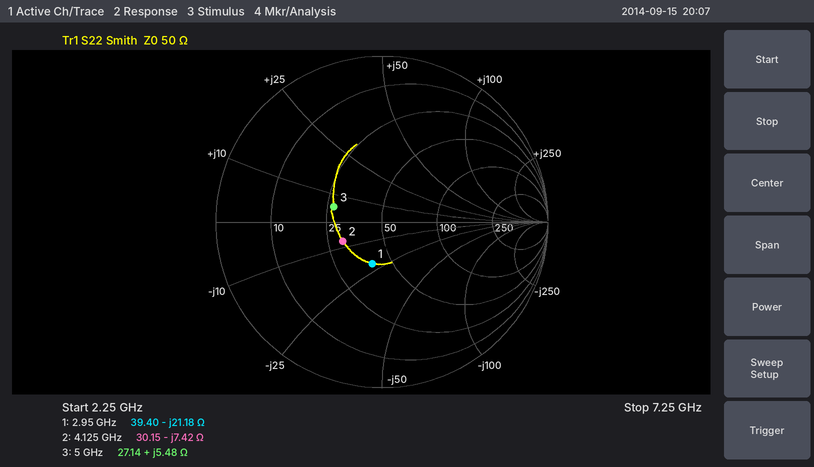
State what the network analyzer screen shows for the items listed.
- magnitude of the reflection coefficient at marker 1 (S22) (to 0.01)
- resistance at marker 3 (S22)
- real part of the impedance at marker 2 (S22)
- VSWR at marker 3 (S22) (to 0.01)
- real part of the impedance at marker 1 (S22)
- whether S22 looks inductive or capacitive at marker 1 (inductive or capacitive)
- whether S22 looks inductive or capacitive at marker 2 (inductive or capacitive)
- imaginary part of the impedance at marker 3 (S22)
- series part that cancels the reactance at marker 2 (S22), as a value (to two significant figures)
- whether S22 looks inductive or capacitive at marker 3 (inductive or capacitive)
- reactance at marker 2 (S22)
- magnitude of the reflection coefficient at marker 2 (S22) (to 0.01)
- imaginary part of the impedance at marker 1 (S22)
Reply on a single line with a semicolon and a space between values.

0.26; 27.14 Ω; 30.15 Ω; 1.87; 39.40 Ω; capacitive; capacitive; +5.48 Ω; 290 pH; inductive; -7.42 Ω; 0.26; -21.18 Ω
